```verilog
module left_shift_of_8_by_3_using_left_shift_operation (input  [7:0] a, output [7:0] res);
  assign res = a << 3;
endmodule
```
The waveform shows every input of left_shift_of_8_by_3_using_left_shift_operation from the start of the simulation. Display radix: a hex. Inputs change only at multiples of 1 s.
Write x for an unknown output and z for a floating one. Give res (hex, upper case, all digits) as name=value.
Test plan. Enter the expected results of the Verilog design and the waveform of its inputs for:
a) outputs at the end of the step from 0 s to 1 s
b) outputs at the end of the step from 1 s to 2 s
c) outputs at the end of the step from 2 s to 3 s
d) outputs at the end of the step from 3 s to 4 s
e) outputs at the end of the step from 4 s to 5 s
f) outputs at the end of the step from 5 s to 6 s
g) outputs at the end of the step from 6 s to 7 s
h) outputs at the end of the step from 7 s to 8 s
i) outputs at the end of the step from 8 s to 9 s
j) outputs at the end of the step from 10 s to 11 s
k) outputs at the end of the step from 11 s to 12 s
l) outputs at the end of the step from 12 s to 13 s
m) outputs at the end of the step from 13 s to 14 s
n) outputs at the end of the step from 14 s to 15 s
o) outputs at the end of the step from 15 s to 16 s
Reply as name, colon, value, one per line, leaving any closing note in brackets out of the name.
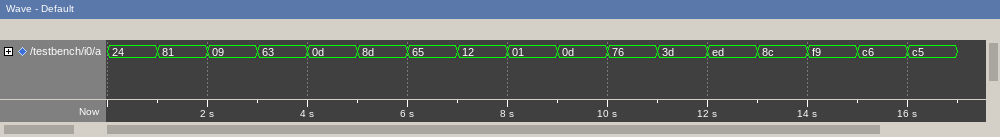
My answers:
outputs at the end of the step from 0 s to 1 s: res=20
outputs at the end of the step from 1 s to 2 s: res=08
outputs at the end of the step from 2 s to 3 s: res=48
outputs at the end of the step from 3 s to 4 s: res=18
outputs at the end of the step from 4 s to 5 s: res=68
outputs at the end of the step from 5 s to 6 s: res=68
outputs at the end of the step from 6 s to 7 s: res=28
outputs at the end of the step from 7 s to 8 s: res=90
outputs at the end of the step from 8 s to 9 s: res=08
outputs at the end of the step from 10 s to 11 s: res=B0
outputs at the end of the step from 11 s to 12 s: res=E8
outputs at the end of the step from 12 s to 13 s: res=68
outputs at the end of the step from 13 s to 14 s: res=60
outputs at the end of the step from 14 s to 15 s: res=C8
outputs at the end of the step from 15 s to 16 s: res=30
